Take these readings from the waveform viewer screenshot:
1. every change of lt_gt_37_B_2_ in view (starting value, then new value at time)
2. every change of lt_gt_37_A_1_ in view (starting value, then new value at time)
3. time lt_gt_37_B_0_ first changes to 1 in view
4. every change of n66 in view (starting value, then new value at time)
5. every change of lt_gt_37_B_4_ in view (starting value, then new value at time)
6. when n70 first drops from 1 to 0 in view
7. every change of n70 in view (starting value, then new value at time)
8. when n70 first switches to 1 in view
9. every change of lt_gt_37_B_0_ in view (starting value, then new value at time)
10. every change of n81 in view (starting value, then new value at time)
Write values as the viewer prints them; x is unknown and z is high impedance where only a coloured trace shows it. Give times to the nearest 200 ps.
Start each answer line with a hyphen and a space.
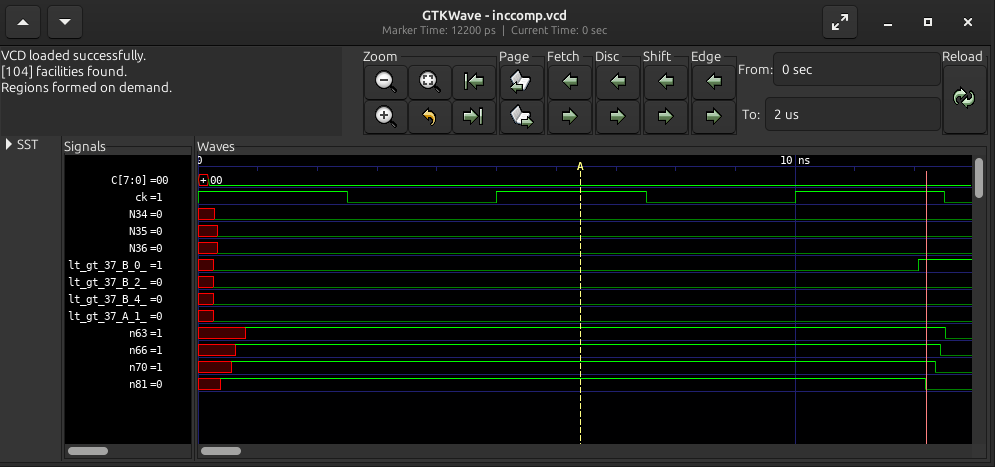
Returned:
- x, 0 at 200 ps
- x, 0 at 200 ps
- 12000 ps
- x, 1 at 600 ps, 0 at 12400 ps
- x, 0 at 200 ps
- 12400 ps
- x, 1 at 600 ps, 0 at 12400 ps
- 600 ps
- x, 0 at 200 ps, 1 at 12000 ps
- x, 1 at 400 ps, 0 at 12200 ps
